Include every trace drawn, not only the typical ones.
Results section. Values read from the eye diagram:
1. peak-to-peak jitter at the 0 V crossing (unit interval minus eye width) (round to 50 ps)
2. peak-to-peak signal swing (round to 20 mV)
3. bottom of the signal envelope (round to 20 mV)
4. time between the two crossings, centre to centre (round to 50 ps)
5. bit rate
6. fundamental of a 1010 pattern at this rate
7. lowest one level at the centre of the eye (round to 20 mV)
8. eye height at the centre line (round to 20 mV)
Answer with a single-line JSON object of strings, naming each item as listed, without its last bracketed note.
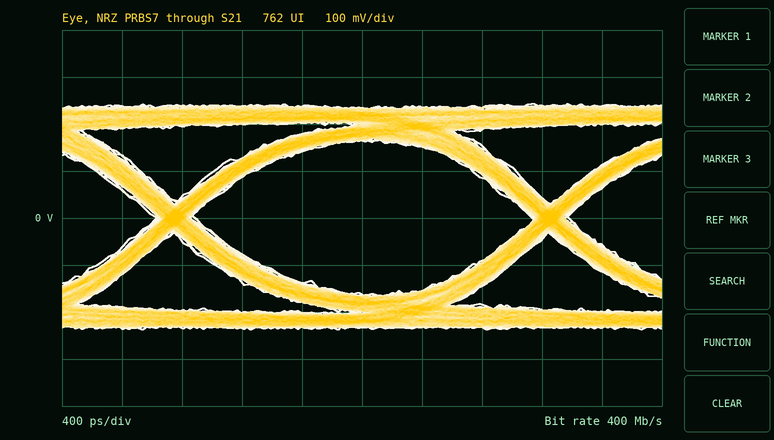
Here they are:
{"peak-to-peak jitter at the 0 V crossing (unit interval minus eye width)": "250 ps", "peak-to-peak signal swing": "480 mV", "bottom of the signal envelope": "-240 mV", "time between the two crossings, centre to centre": "2.50 ns", "bit rate": "400 Mb/s", "fundamental of a 1010 pattern at this rate": "200 MHz", "lowest one level at the centre of the eye": "160 mV", "eye height at the centre line": "320 mV"}
